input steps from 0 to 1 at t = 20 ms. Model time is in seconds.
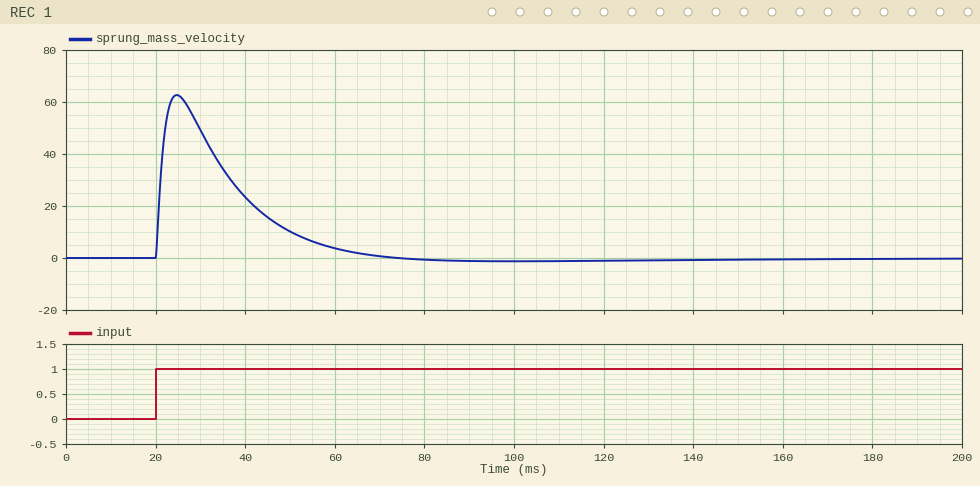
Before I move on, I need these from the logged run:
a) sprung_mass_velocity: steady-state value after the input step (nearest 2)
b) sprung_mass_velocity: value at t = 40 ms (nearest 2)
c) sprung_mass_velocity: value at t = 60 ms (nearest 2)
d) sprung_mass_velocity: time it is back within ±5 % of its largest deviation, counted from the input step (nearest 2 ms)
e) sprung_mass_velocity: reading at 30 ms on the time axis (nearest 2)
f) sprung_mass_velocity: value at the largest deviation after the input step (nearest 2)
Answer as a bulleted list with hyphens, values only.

- 0
- 24
- 4
- 42 ms
- 50
- 62
